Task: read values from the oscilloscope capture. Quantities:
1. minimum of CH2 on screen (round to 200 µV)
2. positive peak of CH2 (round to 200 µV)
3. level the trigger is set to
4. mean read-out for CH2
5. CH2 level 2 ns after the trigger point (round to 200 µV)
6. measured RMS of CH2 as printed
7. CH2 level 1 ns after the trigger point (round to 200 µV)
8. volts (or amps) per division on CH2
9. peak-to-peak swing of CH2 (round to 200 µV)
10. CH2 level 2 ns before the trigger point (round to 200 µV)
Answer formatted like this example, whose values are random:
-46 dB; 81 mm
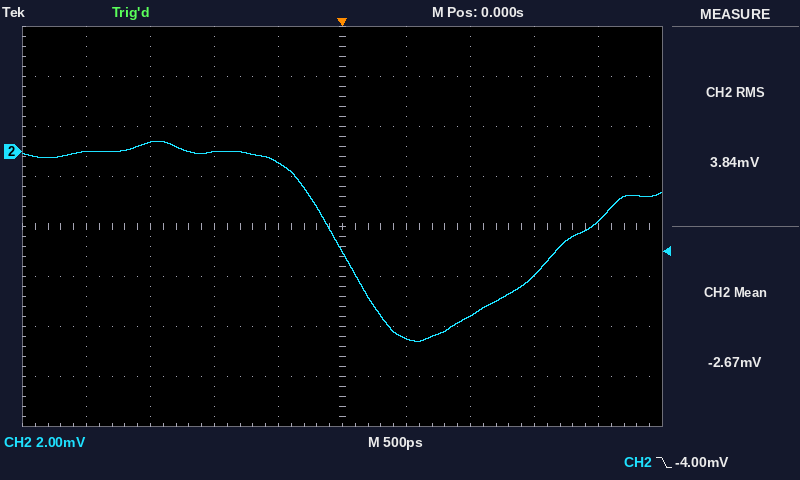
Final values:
-7.6 mV; 400 µV; -4.00 mV; -2.67 mV; -2.8 mV; 3.84 mV; -6.6 mV; 2 mV; 8.0 mV; 0.0 mV
